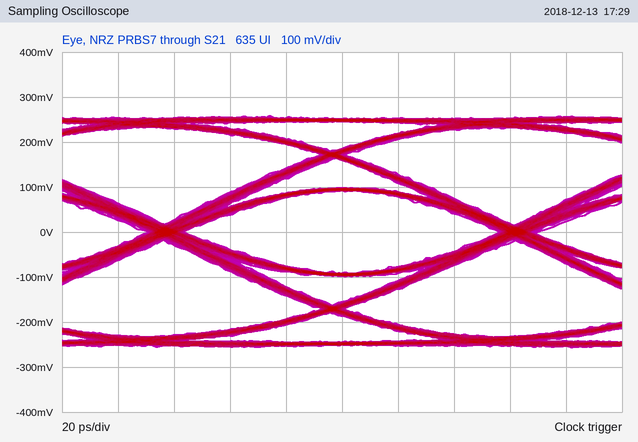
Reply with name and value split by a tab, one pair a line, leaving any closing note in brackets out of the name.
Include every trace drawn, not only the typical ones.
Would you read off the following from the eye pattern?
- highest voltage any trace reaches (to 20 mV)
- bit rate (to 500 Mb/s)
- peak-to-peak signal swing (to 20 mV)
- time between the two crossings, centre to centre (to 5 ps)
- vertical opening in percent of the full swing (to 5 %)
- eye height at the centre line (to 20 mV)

highest voltage any trace reaches	260 mV
bit rate	8.0 Gb/s
peak-to-peak signal swing	520 mV
time between the two crossings, centre to centre	125 ps
vertical opening in percent of the full swing	35 %
eye height at the centre line	180 mV
